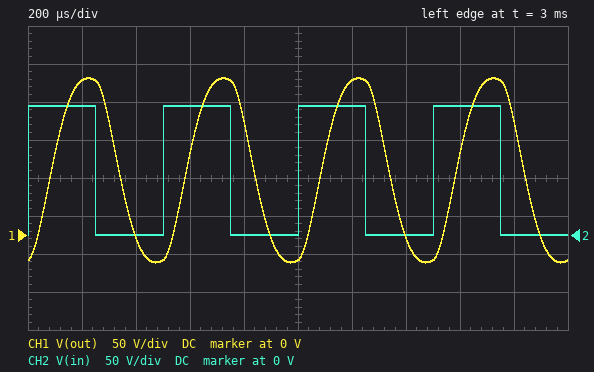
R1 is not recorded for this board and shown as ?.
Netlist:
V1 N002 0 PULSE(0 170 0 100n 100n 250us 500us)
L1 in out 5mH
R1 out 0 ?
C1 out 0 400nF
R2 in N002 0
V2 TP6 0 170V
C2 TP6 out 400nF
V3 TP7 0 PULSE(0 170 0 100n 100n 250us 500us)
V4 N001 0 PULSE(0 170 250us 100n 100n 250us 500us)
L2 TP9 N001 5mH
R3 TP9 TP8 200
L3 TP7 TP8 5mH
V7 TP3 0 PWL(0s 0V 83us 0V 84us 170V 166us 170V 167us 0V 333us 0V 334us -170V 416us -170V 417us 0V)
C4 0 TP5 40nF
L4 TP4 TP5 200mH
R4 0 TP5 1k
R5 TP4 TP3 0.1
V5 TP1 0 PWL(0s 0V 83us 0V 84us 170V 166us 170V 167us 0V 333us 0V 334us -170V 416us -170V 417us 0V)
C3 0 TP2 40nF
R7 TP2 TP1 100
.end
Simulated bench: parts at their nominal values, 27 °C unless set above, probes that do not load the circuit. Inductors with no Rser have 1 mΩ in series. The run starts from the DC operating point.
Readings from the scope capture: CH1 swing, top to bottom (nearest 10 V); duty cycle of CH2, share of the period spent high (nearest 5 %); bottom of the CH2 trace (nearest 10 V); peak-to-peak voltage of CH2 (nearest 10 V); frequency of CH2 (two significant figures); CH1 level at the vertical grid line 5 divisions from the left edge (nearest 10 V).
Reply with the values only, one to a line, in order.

240 V
50 %
0 V
170 V
2.0 kHz
-30 V
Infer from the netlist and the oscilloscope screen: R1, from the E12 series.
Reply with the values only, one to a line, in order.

82 Ω
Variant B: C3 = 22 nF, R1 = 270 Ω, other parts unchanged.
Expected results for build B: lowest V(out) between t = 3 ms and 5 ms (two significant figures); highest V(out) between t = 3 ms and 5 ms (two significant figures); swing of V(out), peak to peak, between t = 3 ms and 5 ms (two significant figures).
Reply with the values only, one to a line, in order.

-160 V
330 V
500 V
